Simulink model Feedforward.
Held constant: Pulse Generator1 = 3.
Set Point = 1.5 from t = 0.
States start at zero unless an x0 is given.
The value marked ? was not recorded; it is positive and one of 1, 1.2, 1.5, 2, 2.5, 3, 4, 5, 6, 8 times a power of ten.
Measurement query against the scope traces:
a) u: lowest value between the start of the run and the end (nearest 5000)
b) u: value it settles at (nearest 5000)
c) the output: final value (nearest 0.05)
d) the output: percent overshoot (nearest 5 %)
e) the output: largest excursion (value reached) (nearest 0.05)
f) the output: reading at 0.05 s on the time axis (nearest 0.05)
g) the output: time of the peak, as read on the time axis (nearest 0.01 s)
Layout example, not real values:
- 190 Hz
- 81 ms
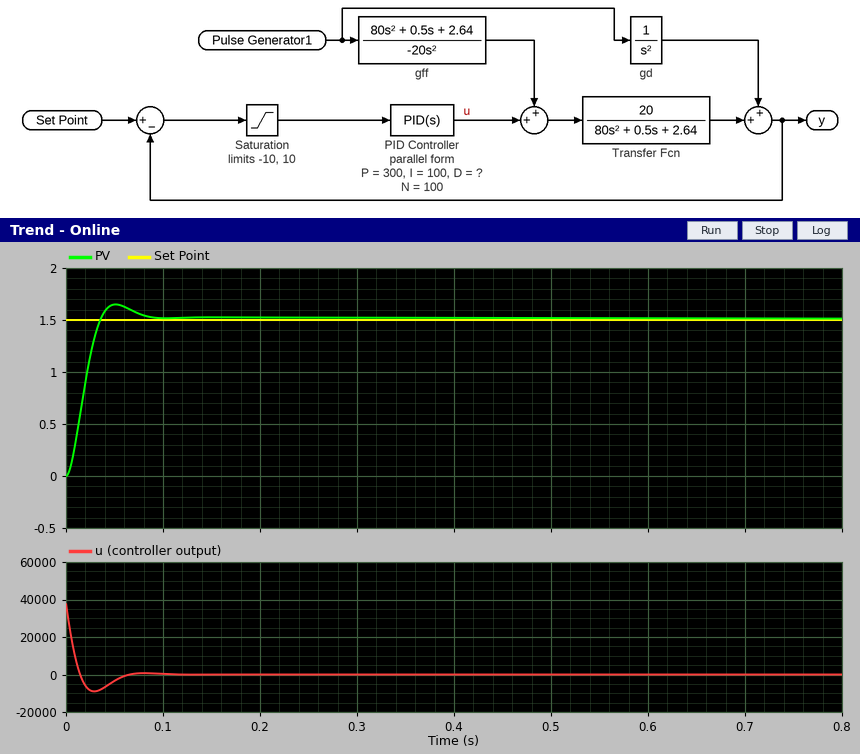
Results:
- -10000
- 0
- 1.50
- 10 %
- 1.65
- 1.65
- 0.05 s
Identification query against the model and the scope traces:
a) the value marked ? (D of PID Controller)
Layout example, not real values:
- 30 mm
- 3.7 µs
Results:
- 250
